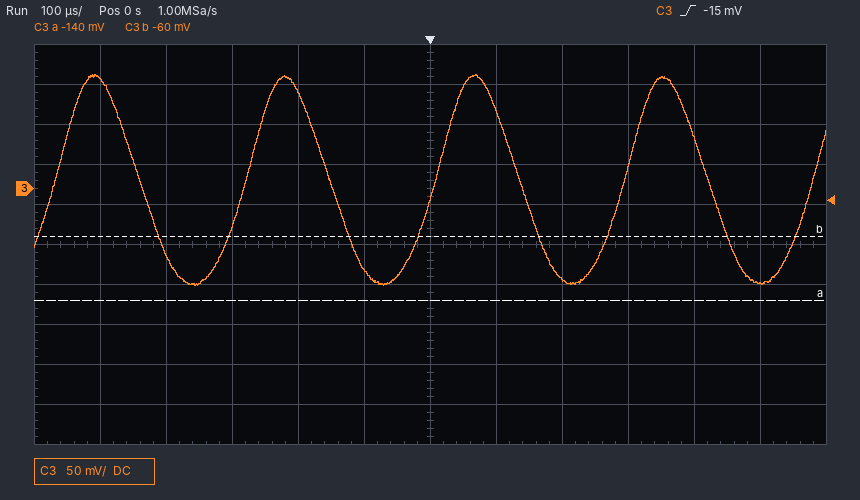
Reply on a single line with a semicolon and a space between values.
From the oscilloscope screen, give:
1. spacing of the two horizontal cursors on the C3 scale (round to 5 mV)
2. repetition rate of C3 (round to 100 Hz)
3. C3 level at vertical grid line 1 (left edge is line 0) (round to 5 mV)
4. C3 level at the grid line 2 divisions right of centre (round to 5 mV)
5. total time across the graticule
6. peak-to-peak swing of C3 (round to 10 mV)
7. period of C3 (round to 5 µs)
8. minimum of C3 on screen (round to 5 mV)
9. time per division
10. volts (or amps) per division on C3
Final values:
80 mV; 3.5 kHz; 135 mV; -115 mV; 1.2 ms; 260 mV; 285 µs; -120 mV; 100 µs; 50 mV
